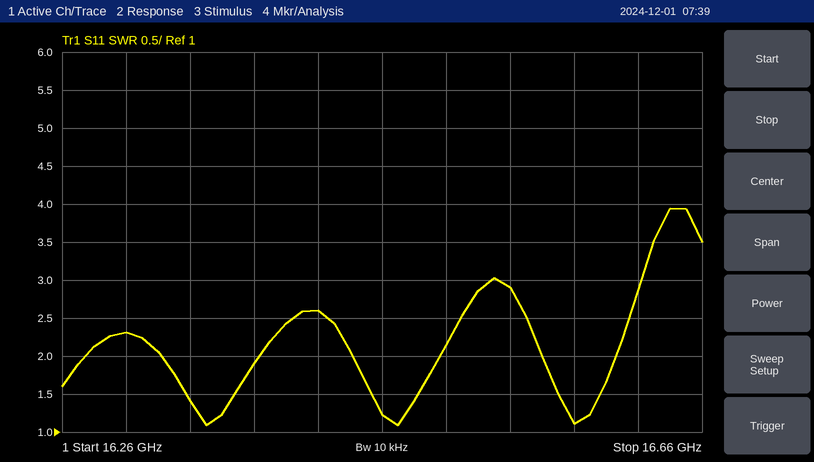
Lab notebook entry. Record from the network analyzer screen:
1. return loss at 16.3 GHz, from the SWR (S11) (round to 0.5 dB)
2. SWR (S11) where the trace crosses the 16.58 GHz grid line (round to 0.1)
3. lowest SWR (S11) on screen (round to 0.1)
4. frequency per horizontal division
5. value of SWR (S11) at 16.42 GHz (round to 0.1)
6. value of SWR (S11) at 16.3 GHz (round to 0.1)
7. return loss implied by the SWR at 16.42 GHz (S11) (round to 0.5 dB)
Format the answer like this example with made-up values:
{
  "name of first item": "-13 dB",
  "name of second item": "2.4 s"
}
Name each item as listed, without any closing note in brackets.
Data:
{
  "return loss at 16.3 GHz, from the SWR (S11)": "8.0 dB",
  "SWR (S11) where the trace crosses the 16.58 GHz grid line": "1.1",
  "lowest SWR (S11) on screen": "1.1",
  "frequency per horizontal division": "40 MHz",
  "value of SWR (S11) at 16.42 GHz": "2.6",
  "value of SWR (S11) at 16.3 GHz": "2.3",
  "return loss implied by the SWR at 16.42 GHz (S11)": "7.0 dB"
}
